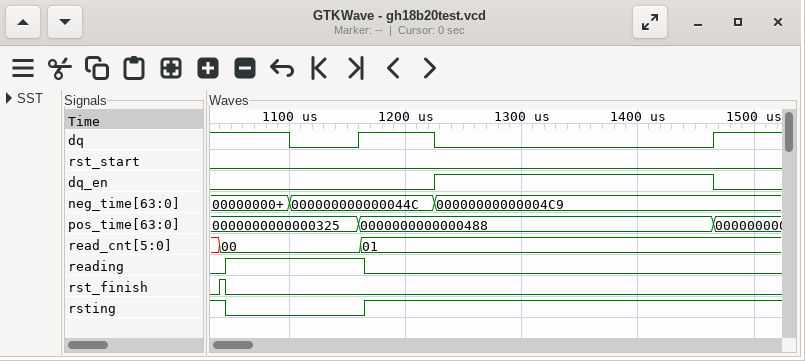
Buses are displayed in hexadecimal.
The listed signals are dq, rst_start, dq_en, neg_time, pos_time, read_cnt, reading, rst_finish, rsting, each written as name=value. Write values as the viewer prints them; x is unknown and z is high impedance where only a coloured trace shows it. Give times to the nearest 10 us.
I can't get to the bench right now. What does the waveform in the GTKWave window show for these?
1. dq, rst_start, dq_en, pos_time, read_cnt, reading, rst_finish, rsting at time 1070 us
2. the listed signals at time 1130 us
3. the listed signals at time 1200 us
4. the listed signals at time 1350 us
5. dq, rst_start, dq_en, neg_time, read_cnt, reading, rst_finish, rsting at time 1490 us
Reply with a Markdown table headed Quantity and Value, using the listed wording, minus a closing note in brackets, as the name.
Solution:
| Quantity | Value |
|---|---|
| dq, rst_start, dq_en, pos_time, read_cnt, reading, rst_finish, rsting at time 1070 us | dq=1, rst_start=0, dq_en=0, pos_time=0000000000000325, read_cnt=00, reading=1, rst_finish=0, rsting=0 |
| the listed signals at time 1130 us | dq=0, rst_start=0, dq_en=0, neg_time=000000000000044C, pos_time=0000000000000325, read_cnt=00, reading=1, rst_finish=0, rsting=0 |
| the listed signals at time 1200 us | dq=1, rst_start=0, dq_en=0, neg_time=000000000000044C, pos_time=0000000000000488, read_cnt=01, reading=0, rst_finish=0, rsting=1 |
| the listed signals at time 1350 us | dq=0, rst_start=0, dq_en=1, neg_time=00000000000004C9, pos_time=0000000000000488, read_cnt=01, reading=0, rst_finish=0, rsting=1 |
| dq, rst_start, dq_en, neg_time, read_cnt, reading, rst_finish, rsting at time 1490 us | dq=1, rst_start=0, dq_en=0, neg_time=00000000000004C9, read_cnt=01, reading=0, rst_finish=0, rsting=1 |
